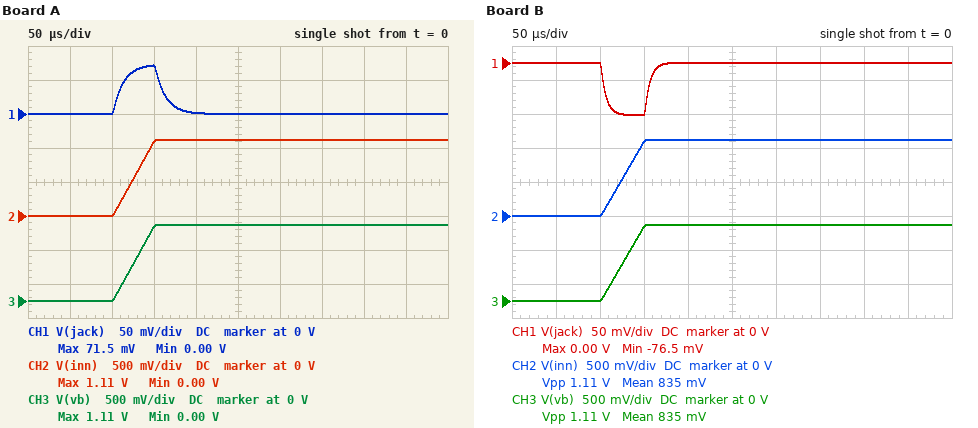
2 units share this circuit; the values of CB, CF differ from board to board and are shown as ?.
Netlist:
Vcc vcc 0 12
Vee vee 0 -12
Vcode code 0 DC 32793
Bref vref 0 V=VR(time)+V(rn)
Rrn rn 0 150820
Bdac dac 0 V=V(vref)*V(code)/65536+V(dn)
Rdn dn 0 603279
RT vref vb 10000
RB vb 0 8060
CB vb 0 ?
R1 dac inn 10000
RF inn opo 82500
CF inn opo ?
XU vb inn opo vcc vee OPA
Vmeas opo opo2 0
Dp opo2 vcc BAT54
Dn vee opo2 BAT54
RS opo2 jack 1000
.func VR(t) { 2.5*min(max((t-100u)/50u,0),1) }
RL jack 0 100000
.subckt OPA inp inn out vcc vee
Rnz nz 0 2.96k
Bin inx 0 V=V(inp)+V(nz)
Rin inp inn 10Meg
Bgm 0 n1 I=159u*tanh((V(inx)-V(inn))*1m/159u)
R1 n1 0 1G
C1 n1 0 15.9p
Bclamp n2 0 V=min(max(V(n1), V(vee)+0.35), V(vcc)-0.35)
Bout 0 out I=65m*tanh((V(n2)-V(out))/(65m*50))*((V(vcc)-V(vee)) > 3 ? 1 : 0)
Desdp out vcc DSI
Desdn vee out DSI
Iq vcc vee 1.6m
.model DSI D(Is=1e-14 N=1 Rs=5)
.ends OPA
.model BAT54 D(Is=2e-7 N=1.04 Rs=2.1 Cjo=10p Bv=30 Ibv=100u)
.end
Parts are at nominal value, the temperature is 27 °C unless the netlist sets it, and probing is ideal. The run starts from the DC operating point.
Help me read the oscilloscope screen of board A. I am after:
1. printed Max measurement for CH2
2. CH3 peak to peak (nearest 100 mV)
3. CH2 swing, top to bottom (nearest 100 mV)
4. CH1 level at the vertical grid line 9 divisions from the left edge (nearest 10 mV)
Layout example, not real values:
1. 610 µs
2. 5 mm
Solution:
1. 1.11 V
2. 1.1 V
3. 1.1 V
4. 0 V
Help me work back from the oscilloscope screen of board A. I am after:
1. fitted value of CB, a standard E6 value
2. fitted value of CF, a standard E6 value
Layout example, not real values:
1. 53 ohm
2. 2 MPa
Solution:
1. 220 pF
2. 150 pF
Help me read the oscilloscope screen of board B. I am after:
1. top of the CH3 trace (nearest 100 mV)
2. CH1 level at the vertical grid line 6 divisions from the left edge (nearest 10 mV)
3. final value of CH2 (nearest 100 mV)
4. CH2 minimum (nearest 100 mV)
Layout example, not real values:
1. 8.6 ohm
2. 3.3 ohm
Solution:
1. 1.1 V
2. 0 V
3. 1.1 V
4. 0 V
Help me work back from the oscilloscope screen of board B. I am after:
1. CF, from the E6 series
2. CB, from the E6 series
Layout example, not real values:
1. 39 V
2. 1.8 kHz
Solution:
1. 68 pF
2. 220 pF
